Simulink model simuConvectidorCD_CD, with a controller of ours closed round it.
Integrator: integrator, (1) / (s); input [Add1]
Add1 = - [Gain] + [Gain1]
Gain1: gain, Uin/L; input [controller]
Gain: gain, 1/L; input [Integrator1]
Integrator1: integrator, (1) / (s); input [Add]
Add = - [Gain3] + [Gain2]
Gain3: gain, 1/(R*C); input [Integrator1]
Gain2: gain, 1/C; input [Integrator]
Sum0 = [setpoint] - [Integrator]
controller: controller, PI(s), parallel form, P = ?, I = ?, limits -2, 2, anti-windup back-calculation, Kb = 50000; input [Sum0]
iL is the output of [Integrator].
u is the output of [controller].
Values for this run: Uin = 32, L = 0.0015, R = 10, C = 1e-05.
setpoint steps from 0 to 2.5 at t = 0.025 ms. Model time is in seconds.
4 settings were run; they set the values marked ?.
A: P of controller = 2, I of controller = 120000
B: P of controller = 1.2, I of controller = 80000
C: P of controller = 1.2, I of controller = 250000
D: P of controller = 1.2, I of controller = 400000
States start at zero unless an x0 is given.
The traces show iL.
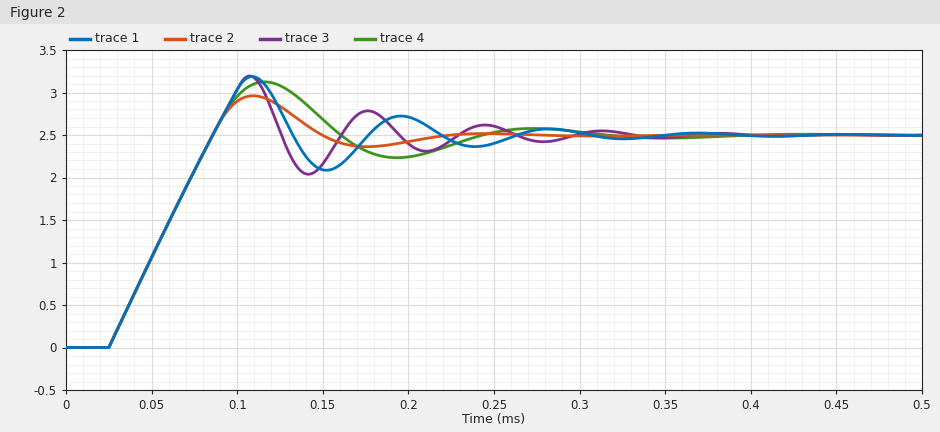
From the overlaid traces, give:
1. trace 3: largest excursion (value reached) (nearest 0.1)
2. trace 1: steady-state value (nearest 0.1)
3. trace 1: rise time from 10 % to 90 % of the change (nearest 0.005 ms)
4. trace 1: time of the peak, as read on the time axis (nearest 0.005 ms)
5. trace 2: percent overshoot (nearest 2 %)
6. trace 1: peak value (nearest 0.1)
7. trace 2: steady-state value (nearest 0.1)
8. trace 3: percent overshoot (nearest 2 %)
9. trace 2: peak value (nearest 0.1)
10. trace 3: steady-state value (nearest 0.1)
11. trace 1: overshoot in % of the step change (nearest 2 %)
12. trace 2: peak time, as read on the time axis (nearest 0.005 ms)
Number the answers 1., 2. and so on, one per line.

1. 3.2
2. 2.5
3. 0.050 ms
4. 0.110 ms
5. 18 %
6. 3.2
7. 2.5
8. 28 %
9. 3.0
10. 2.5
11. 28 %
12. 0.110 ms
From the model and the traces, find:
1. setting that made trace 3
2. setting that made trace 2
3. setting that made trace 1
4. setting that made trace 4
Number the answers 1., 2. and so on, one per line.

1. D
2. A
3. C
4. B
